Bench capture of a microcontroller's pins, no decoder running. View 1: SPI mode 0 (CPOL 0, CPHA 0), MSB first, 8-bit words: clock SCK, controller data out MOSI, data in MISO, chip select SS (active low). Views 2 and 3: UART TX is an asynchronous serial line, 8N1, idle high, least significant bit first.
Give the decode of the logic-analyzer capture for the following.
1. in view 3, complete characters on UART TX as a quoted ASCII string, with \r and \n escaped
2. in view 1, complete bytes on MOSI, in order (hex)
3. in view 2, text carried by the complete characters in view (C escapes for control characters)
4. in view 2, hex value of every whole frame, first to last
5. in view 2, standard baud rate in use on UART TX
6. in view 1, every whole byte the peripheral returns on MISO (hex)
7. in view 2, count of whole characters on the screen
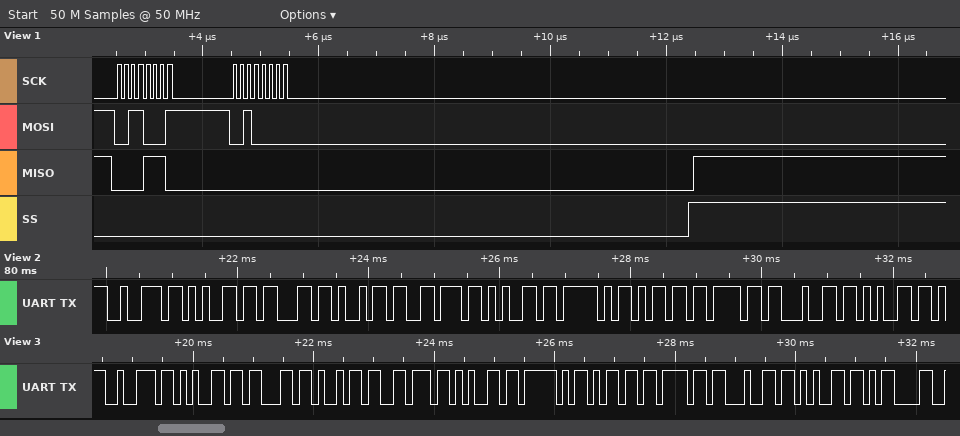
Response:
"recive_mode\r"
31 20
"recive_mode"
0x72 0x65 0x63 0x69 0x76 0x65 0x5F 0x6D 0x6F 0x64 0x65
9600 baud
0E 00
11
